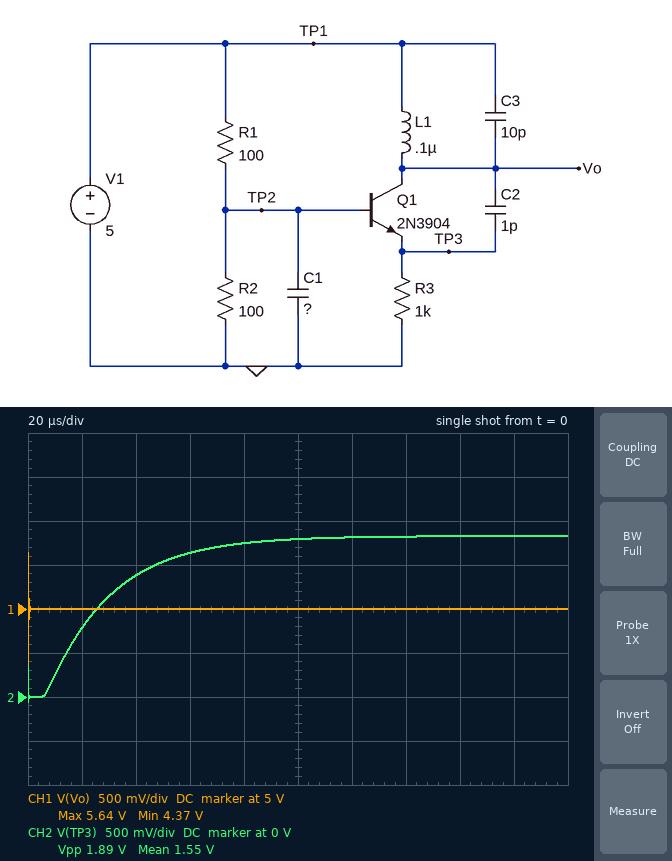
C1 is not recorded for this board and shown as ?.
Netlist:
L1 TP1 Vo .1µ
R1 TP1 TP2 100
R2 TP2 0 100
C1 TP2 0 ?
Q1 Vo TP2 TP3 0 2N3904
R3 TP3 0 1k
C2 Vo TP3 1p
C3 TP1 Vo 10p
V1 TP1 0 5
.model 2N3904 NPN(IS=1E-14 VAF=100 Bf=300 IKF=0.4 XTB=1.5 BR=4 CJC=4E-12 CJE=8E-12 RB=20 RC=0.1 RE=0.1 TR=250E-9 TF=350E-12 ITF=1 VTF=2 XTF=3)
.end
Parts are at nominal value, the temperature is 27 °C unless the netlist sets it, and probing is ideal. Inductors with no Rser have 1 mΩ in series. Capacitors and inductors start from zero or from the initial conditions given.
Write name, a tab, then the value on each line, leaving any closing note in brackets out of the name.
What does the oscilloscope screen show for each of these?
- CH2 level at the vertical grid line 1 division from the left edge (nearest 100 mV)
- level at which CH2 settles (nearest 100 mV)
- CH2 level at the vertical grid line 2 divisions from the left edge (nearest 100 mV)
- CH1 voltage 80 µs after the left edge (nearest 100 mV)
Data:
CH2 level at the vertical grid line 1 division from the left edge	800 mV
level at which CH2 settles	1.8 V
CH2 level at the vertical grid line 2 divisions from the left edge	1.4 V
CH1 voltage 80 µs after the left edge	5.0 V
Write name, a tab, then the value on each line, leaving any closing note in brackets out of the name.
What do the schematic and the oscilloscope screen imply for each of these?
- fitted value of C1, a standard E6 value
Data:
fitted value of C1, a standard E6 value	470 nF
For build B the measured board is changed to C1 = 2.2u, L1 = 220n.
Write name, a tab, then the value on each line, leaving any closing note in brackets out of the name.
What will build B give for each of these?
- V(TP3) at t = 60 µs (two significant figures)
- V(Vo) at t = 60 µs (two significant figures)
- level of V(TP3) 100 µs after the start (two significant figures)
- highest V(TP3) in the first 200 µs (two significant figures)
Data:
V(TP3) at t = 60 µs	420 mV
V(Vo) at t = 60 µs	5.0 V
level of V(TP3) 100 µs after the start	840 mV
highest V(TP3) in the first 200 µs	1.4 V
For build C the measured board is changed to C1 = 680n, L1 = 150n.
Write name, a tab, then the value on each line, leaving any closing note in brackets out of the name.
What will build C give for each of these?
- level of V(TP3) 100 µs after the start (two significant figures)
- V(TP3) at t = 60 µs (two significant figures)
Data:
level of V(TP3) 100 µs after the start	1.7 V
V(TP3) at t = 60 µs	1.4 V
